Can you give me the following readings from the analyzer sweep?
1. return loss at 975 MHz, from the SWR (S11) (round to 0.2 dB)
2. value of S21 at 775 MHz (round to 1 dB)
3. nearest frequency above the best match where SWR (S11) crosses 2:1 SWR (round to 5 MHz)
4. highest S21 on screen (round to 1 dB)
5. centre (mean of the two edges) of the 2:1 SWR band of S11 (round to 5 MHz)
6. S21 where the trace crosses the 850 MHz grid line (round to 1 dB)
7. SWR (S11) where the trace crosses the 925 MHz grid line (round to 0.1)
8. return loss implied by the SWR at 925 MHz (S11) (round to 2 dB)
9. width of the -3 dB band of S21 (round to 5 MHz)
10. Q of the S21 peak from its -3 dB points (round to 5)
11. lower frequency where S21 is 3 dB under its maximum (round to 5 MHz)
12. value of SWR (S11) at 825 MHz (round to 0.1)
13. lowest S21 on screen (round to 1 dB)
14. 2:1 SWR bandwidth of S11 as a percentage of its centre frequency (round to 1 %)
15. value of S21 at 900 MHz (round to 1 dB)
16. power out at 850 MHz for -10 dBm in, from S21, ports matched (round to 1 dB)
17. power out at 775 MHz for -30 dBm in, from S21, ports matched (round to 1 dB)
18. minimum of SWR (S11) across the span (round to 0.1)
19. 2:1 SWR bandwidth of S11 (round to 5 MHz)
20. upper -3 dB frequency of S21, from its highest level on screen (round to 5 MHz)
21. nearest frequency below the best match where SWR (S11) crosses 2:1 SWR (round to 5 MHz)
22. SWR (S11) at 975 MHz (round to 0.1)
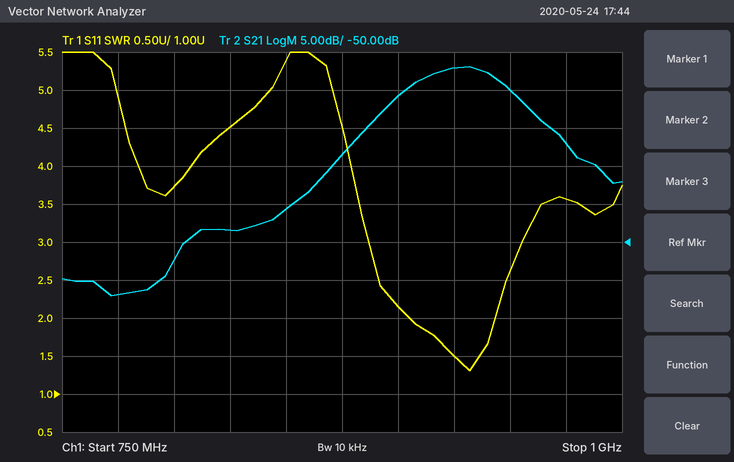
5.0 dB
-57 dB
945 MHz
-27 dB
925 MHz
-46 dB
1.5
14 dB
45 MHz
20
905 MHz
4.5
-57 dB
4 %
-31 dB
-56 dBm
-87 dBm
1.3
40 MHz
950 MHz
905 MHz
3.6
